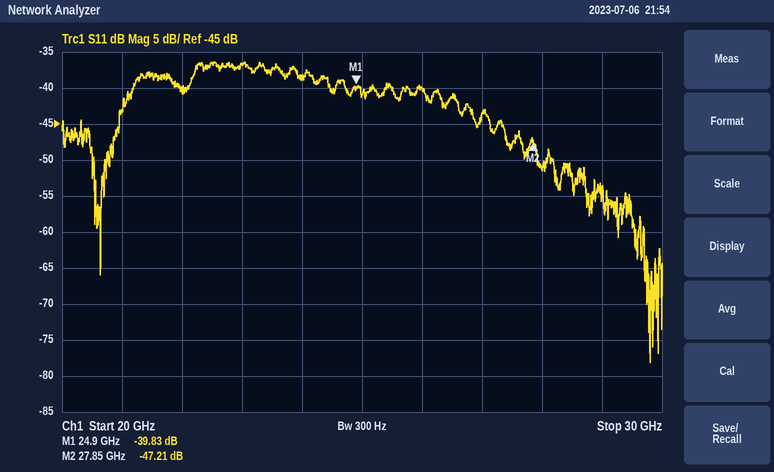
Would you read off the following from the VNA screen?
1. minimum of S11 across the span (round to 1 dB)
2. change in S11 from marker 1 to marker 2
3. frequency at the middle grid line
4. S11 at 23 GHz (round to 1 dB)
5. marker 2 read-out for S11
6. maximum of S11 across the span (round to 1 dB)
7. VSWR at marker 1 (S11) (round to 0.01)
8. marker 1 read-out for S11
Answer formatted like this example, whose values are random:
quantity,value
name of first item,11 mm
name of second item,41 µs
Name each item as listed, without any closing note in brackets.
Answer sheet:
quantity,value
minimum of S11 across the span,-78 dB
change in S11 from marker 1 to marker 2,-7.38 dB
frequency at the middle grid line,25 GHz
S11 at 23 GHz,-37 dB
marker 2 read-out for S11,-47.21 dB
maximum of S11 across the span,-36 dB
VSWR at marker 1 (S11),1.02
marker 1 read-out for S11,-39.83 dB
